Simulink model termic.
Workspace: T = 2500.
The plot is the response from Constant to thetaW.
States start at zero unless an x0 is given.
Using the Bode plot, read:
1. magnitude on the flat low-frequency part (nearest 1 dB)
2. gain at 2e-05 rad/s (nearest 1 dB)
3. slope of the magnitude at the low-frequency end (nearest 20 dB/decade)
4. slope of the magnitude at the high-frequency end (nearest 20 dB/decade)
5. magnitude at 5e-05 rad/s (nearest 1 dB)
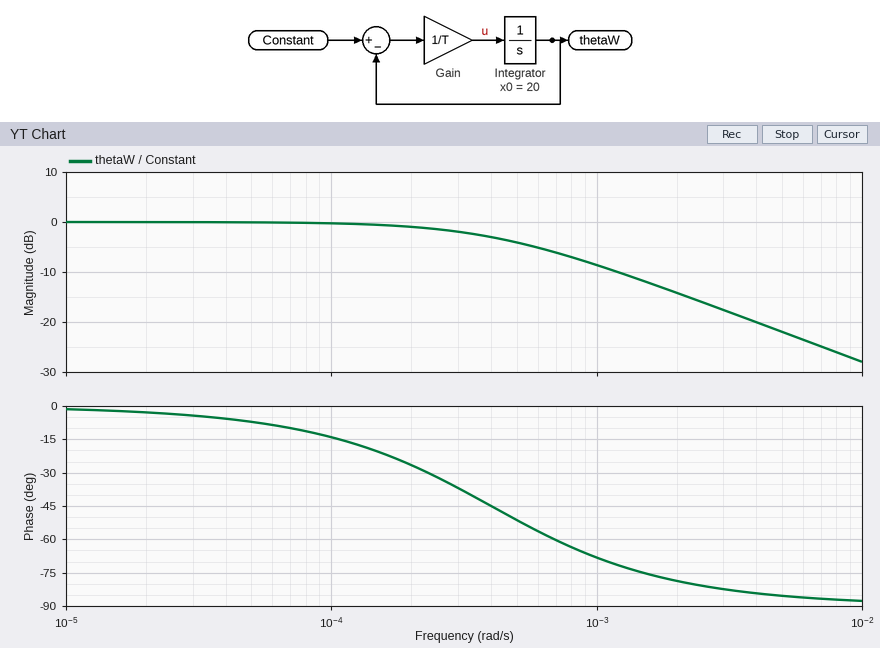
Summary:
0 dB
0 dB
0 dB/decade
-20 dB/decade
0 dB
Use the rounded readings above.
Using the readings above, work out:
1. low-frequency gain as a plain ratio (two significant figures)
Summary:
1.0
